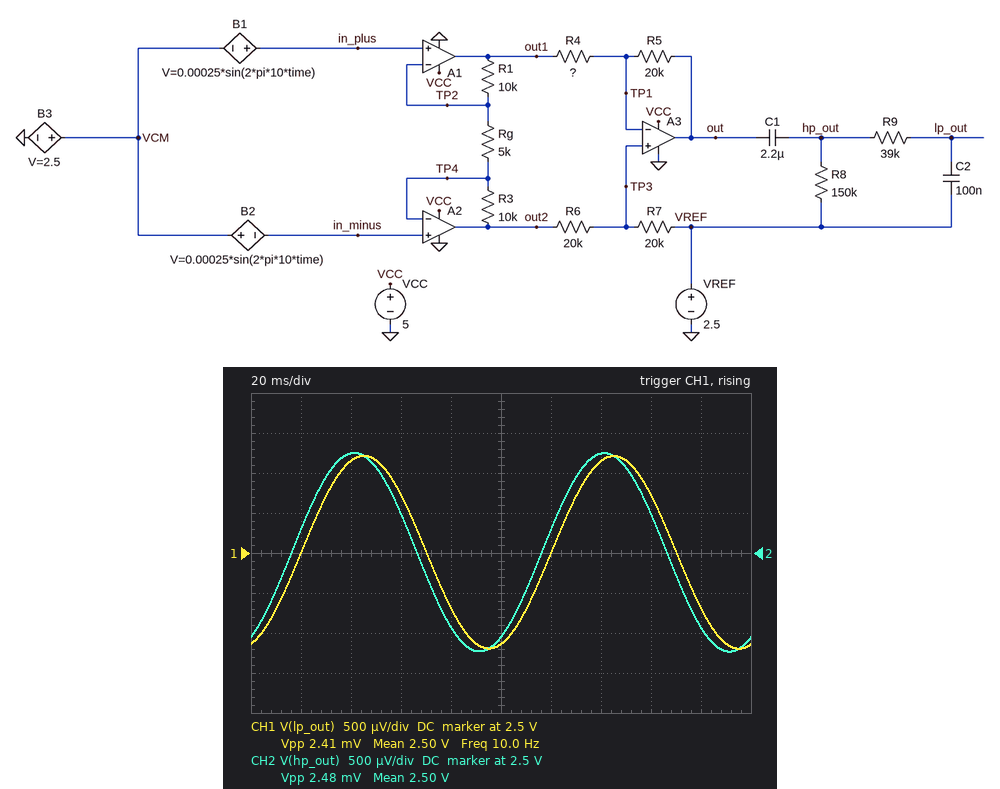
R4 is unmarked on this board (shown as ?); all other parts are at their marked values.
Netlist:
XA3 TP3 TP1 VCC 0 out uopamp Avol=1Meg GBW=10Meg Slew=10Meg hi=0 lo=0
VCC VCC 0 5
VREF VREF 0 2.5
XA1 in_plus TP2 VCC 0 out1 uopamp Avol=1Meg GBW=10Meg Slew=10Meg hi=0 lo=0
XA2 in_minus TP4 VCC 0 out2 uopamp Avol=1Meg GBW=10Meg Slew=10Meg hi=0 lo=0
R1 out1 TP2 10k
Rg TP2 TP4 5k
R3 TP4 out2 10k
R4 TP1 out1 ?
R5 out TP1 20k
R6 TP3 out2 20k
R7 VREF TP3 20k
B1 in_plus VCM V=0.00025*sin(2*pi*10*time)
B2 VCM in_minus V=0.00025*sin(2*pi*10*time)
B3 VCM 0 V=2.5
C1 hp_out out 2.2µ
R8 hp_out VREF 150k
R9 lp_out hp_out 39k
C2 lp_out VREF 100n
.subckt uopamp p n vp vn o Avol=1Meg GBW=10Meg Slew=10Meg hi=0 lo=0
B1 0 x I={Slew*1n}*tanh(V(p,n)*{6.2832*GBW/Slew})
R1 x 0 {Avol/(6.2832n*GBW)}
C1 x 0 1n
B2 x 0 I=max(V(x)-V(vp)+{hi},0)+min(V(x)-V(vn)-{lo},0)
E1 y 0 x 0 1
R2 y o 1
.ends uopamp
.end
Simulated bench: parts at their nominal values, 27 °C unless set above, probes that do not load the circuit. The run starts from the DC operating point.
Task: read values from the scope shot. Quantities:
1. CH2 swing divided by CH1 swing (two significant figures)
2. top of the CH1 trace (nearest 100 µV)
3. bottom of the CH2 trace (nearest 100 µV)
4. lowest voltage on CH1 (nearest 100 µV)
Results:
1.0
2.5012 V
2.4988 V
2.4988 V
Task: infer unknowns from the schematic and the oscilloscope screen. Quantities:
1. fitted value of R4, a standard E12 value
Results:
56 kΩ
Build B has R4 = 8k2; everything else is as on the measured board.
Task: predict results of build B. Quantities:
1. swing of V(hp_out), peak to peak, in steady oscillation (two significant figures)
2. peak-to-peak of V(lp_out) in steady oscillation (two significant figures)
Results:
10 mV
9.7 mV
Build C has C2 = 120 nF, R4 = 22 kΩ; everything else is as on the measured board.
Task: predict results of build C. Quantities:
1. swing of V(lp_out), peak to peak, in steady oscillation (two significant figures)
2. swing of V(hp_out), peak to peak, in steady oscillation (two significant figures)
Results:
4.3 mV
4.4 mV
